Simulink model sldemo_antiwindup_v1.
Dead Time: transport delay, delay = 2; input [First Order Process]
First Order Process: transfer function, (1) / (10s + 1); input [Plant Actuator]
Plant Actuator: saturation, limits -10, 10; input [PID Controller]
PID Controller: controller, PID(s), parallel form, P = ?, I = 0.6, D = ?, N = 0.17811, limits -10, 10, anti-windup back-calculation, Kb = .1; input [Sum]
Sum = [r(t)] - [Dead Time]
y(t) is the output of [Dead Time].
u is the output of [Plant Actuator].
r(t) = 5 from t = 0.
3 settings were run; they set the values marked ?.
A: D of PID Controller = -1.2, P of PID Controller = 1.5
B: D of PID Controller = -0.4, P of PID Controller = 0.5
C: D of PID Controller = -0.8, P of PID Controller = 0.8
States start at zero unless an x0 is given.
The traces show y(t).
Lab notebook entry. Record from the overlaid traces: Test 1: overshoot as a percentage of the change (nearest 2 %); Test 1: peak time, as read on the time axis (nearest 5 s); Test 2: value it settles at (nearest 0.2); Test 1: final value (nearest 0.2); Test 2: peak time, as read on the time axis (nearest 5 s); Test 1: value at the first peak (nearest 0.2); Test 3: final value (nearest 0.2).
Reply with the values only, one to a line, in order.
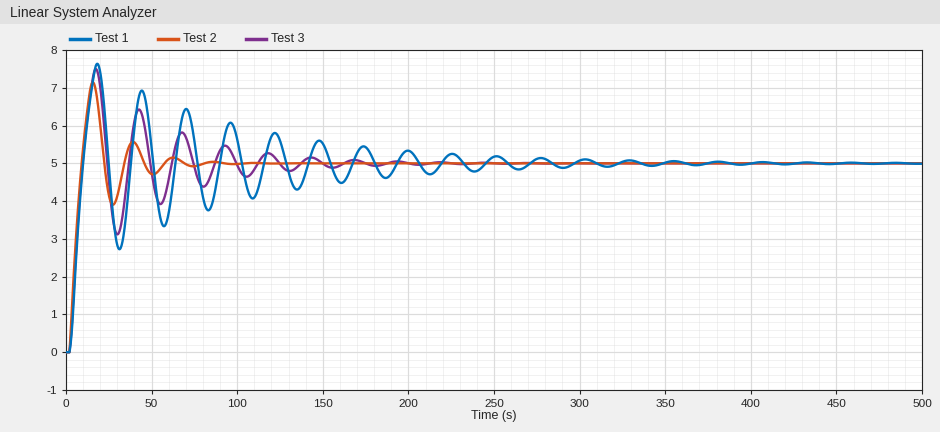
52 %
20 s
5.0
5.0
15 s
7.6
5.0
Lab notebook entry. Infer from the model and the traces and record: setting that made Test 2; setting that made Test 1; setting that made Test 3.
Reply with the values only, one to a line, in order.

A
B
C
